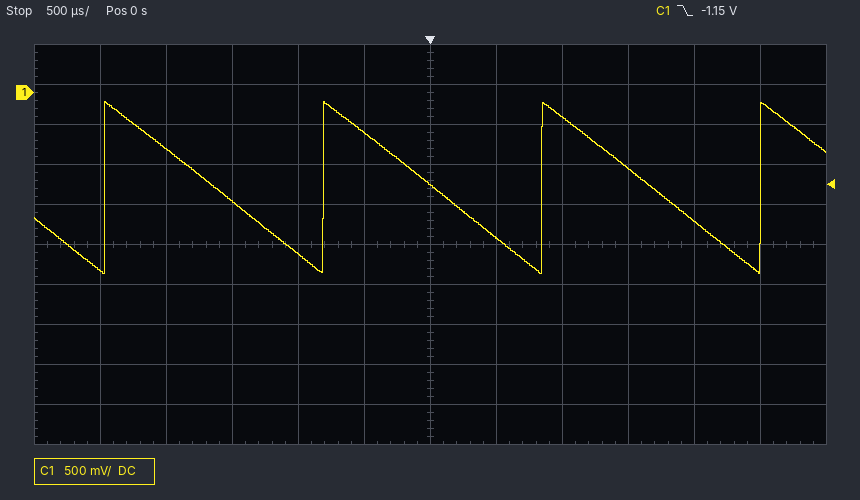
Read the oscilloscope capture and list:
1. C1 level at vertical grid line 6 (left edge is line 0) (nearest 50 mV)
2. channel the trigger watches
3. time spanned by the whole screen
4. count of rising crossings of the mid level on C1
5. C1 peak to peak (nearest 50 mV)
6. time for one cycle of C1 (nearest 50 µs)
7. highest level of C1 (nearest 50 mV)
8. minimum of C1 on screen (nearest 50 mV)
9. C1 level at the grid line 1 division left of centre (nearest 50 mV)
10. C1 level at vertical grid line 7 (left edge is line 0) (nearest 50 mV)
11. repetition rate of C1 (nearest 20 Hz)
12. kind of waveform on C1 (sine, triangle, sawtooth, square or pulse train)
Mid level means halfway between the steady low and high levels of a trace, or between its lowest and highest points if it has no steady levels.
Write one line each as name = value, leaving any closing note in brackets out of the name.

C1 level at vertical grid line 6 (left edge is line 0) = -1.15 V
channel the trigger watches = C1
time spanned by the whole screen = 6 ms
count of rising crossings of the mid level on C1 = 4
C1 peak to peak = 2.15 V
time for one cycle of C1 = 1.65 ms
highest level of C1 = -100 mV
minimum of C1 on screen = -2.25 V
C1 level at the grid line 1 division left of centre = -500 mV
C1 level at vertical grid line 7 (left edge is line 0) = -1.80 V
repetition rate of C1 = 600 Hz
kind of waveform on C1 = sawtooth
